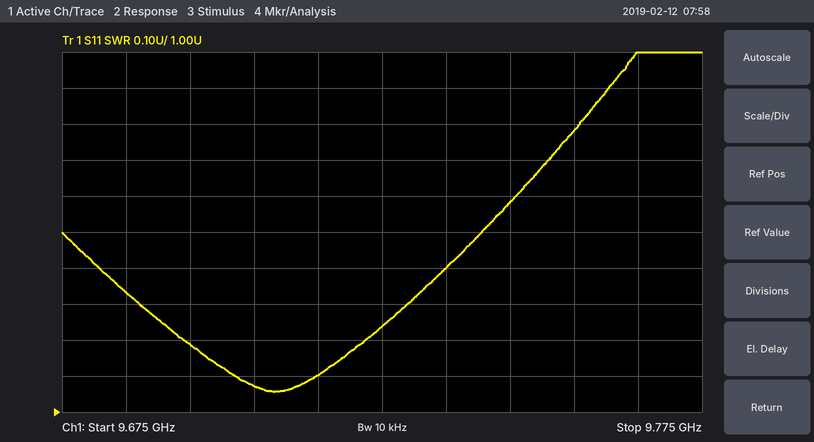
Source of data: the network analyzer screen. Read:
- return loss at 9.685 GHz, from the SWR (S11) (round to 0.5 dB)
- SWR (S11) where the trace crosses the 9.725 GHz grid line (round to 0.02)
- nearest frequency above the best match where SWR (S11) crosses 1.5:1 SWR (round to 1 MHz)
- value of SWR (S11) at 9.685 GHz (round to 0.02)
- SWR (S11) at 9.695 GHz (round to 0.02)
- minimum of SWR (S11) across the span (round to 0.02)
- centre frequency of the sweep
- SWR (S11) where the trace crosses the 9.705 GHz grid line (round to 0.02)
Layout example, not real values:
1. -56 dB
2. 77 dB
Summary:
1. 17.0 dB
2. 1.24
3. 9.741 GHz
4. 1.34
5. 1.18
6. 1.06
7. 9.725 GHz
8. 1.08
